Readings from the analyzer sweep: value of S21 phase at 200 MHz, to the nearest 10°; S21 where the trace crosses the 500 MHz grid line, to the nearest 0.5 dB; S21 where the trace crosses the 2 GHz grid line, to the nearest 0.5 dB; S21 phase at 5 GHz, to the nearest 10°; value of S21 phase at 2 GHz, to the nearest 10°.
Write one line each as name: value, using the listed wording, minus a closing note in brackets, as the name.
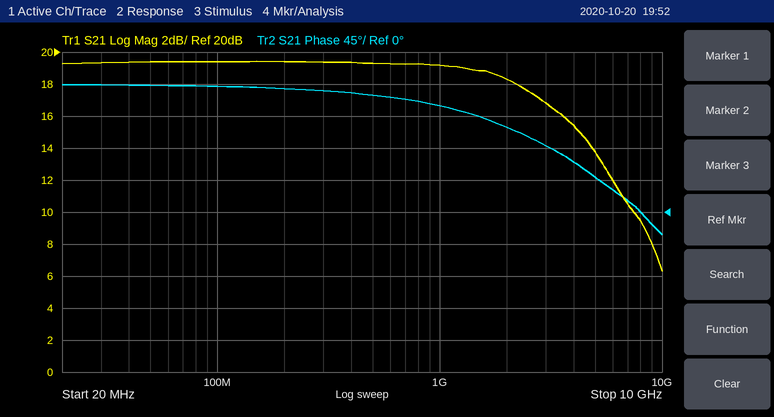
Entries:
value of S21 phase at 200 MHz, to the nearest 10°: 170°
S21 where the trace crosses the 500 MHz grid line, to the nearest 0.5 dB: 19.5 dB
S21 where the trace crosses the 2 GHz grid line, to the nearest 0.5 dB: 18.5 dB
S21 phase at 5 GHz, to the nearest 10°: 50°
value of S21 phase at 2 GHz, to the nearest 10°: 120°
